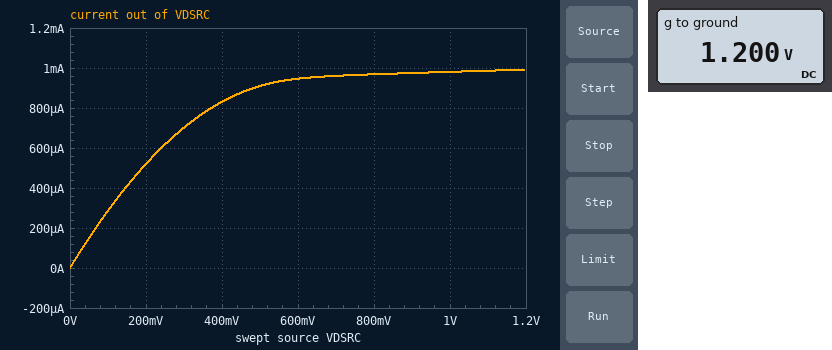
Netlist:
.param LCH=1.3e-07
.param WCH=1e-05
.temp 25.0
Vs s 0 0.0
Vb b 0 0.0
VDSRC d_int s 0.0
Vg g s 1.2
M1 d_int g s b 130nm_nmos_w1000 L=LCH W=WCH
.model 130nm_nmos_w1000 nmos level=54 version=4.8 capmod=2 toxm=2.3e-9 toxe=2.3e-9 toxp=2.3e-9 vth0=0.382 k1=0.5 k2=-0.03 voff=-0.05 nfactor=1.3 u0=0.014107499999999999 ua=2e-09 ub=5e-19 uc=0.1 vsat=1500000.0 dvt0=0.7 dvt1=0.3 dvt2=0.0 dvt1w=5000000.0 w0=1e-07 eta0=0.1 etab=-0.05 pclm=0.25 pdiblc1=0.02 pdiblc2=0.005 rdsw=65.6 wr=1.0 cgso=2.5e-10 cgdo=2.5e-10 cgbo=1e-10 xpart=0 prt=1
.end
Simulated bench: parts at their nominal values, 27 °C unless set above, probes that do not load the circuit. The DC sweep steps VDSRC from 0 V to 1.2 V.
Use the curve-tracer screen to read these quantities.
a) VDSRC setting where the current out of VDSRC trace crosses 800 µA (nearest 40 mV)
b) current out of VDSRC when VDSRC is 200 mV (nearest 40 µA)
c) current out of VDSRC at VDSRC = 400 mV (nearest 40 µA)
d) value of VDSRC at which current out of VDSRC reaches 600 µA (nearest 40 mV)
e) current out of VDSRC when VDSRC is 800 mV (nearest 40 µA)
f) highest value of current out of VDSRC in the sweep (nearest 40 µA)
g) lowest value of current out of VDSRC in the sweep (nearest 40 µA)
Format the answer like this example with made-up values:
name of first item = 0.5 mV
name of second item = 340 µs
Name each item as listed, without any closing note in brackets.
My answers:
VDSRC setting where the current out of VDSRC trace crosses 800 µA = 360 mV
current out of VDSRC when VDSRC is 200 mV = 520 µA
current out of VDSRC at VDSRC = 400 mV = 840 µA
value of VDSRC at which current out of VDSRC reaches 600 µA = 240 mV
current out of VDSRC when VDSRC is 800 mV = 960 µA
highest value of current out of VDSRC in the sweep = 1.00 mA
lowest value of current out of VDSRC in the sweep = 0 A
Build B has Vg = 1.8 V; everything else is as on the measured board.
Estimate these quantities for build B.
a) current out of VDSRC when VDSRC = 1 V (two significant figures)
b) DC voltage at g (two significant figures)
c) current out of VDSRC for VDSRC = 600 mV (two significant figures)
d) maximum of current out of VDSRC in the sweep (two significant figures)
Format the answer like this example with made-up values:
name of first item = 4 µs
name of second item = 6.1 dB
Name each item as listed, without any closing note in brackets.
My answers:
current out of VDSRC when VDSRC = 1 V = 2.8 mA
DC voltage at g = 1.8 V
current out of VDSRC for VDSRC = 600 mV = 2.2 mA
maximum of current out of VDSRC in the sweep = 2.9 mA
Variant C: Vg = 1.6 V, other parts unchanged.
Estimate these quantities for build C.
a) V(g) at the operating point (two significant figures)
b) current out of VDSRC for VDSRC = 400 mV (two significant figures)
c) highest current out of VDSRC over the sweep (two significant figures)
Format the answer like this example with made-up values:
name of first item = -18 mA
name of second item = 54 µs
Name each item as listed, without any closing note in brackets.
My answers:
V(g) at the operating point = 1.6 V
current out of VDSRC for VDSRC = 400 mV = 1.4 mA
highest current out of VDSRC over the sweep = 2.2 mA
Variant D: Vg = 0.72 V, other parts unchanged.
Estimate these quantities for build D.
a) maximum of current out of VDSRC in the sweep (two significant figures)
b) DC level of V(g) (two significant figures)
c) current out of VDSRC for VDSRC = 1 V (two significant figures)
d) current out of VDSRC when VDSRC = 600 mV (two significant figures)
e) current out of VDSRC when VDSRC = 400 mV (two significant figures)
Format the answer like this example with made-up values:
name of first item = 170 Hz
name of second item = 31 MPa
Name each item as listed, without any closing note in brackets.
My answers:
maximum of current out of VDSRC in the sweep = 42 µA
DC level of V(g) = 720 mV
current out of VDSRC for VDSRC = 1 V = 41 µA
current out of VDSRC when VDSRC = 600 mV = 37 µA
current out of VDSRC when VDSRC = 400 mV = 36 µA
